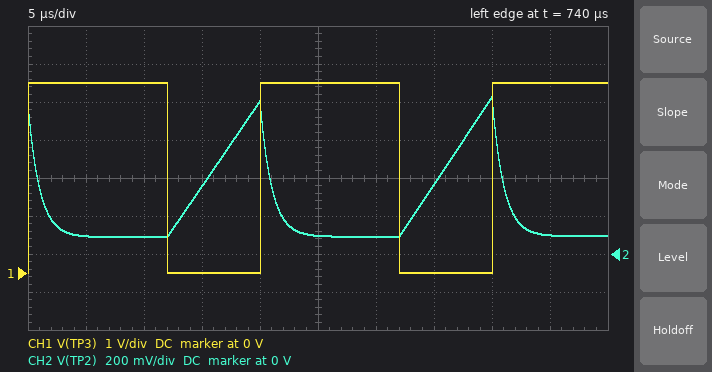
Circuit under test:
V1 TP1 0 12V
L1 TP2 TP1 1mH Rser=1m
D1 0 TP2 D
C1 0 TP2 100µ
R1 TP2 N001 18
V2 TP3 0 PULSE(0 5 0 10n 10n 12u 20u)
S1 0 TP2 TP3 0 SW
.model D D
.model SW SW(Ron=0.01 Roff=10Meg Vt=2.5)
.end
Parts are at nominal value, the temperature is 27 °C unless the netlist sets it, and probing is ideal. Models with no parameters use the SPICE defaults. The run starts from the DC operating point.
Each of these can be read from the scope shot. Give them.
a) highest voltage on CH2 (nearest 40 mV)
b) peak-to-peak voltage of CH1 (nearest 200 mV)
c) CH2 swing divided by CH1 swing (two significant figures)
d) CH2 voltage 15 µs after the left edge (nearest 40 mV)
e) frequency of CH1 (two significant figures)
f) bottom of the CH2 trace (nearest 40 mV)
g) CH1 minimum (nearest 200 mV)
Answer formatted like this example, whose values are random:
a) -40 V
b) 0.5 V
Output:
a) 840 mV
b) 5.0 V
c) 0.15
d) 360 mV
e) 50 kHz
f) 80 mV
g) 0 V
